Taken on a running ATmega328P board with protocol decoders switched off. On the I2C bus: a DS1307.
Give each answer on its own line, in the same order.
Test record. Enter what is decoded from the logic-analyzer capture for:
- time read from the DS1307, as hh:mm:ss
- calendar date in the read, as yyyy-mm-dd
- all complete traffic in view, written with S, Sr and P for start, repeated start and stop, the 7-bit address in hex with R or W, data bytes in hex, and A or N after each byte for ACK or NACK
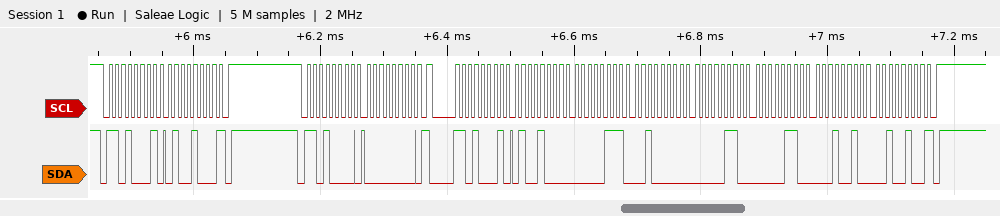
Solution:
20:07:48
2024-12-06
S 68R A 48 N P S 68W A 00 A Sr 68R A 48 A 07 A 20 A 06 A 06 A 12 A 24 N P
